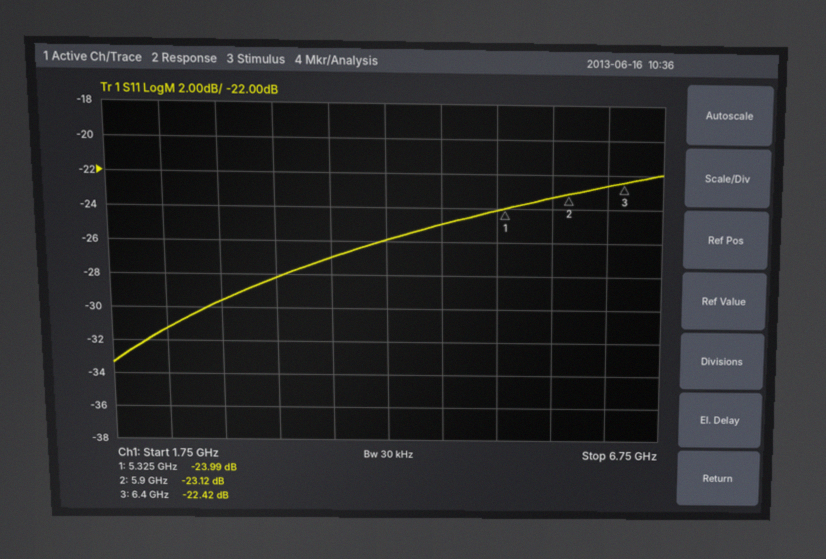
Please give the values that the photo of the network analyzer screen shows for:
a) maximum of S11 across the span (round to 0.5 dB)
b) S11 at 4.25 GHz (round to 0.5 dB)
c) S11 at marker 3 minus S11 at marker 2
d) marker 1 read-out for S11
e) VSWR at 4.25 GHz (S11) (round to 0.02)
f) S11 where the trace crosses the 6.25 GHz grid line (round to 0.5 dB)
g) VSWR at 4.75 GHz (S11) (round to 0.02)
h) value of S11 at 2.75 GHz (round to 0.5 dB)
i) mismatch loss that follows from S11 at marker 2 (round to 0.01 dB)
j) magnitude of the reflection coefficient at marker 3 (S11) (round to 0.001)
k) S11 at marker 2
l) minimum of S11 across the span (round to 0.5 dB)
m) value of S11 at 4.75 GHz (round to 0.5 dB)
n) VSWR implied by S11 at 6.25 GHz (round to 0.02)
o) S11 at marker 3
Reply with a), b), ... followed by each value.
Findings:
a) -22.0 dB
b) -26.0 dB
c) 0.70 dB
d) -23.99 dB
e) 1.10
f) -22.5 dB
g) 1.12
h) -29.5 dB
i) 0.02 dB
j) 0.076
k) -23.12 dB
l) -33.5 dB
m) -25.0 dB
n) 1.16
o) -22.42 dB
